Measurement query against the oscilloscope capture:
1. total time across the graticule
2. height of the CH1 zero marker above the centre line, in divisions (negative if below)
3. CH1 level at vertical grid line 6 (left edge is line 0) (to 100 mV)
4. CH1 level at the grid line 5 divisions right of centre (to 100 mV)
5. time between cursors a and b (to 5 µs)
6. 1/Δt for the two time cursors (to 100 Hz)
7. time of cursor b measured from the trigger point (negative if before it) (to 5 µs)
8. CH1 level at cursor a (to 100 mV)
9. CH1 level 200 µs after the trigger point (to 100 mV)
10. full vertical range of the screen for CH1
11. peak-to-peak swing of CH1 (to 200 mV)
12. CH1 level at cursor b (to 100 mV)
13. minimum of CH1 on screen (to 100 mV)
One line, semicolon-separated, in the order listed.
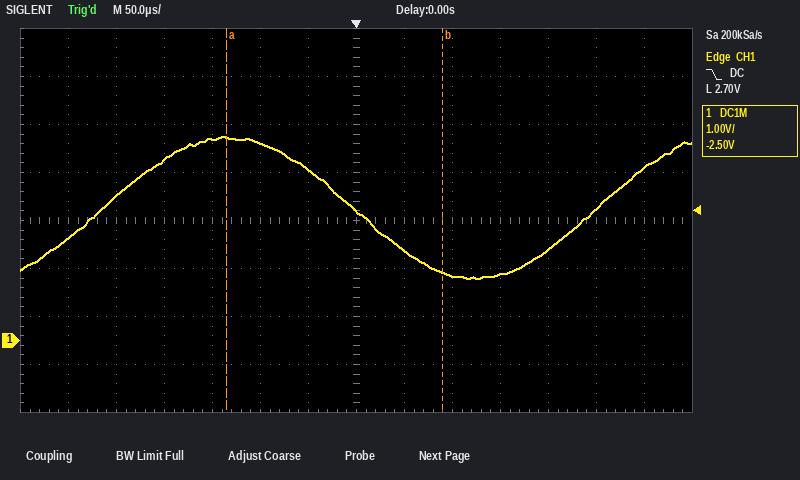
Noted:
700 µs; -2.5 div; 3.6 V; 2.7 V; 225 µs; 4.4 kHz; +90 µs; 4.2 V; 1.9 V; 8 V; 3.0 V; 1.4 V; 1.3 V
